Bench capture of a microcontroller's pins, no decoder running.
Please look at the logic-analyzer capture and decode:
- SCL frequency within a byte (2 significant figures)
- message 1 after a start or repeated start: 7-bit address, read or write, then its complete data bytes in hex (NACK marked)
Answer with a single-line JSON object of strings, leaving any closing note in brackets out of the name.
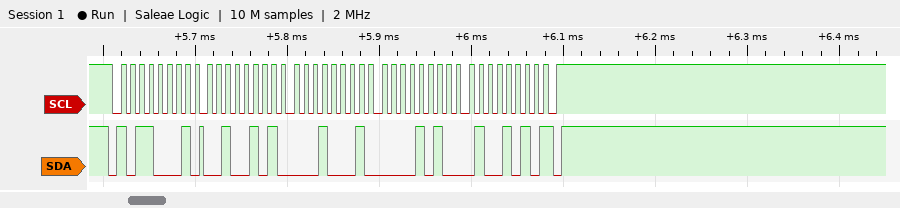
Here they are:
{"SCL frequency within a byte": "100 kHz", "message 1 after a start or repeated start: 7-bit address, read or write, then its complete data bytes in hex": "0x58 read: 25 11 0A 4A NACK"}
